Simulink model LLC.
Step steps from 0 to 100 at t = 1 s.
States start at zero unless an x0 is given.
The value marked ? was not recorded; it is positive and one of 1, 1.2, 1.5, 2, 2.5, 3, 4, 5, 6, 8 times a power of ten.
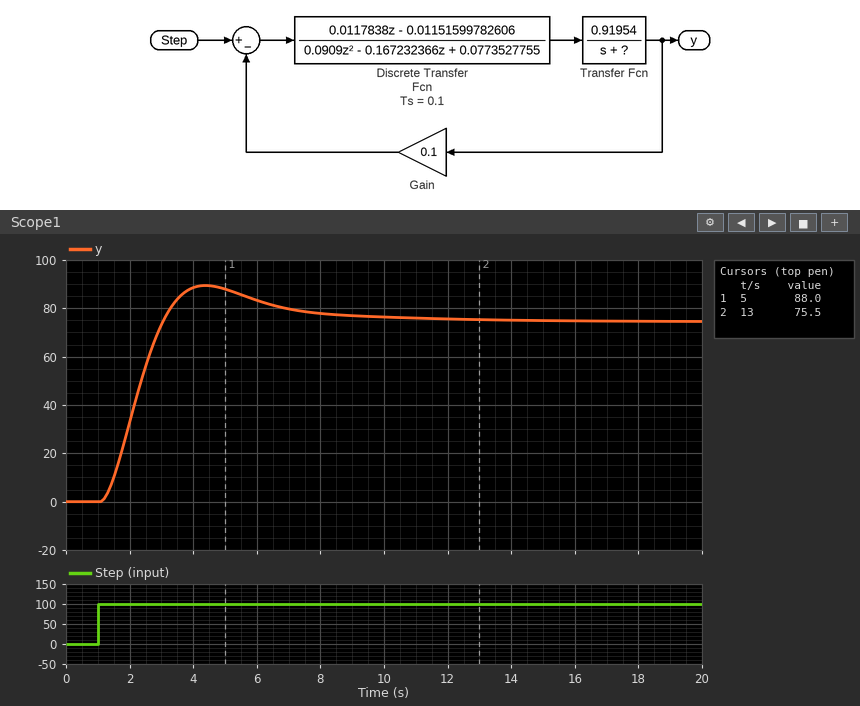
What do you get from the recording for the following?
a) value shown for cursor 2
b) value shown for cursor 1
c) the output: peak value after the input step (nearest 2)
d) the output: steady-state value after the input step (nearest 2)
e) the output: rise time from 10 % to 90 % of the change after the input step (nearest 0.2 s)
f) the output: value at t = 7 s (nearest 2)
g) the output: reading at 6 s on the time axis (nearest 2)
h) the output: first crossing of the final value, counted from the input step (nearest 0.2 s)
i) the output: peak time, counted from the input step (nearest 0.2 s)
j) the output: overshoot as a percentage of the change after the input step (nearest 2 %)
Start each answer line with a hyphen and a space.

- 75.5
- 88.0
- 90
- 74
- 1.4 s
- 80
- 84
- 2.0 s
- 3.4 s
- 20 %
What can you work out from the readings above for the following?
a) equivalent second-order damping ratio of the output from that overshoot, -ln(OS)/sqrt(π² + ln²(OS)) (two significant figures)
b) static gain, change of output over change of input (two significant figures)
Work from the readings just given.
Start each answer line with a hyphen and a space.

- 0.46
- 0.74
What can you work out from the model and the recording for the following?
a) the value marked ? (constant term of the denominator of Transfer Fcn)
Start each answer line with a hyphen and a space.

- 0.3
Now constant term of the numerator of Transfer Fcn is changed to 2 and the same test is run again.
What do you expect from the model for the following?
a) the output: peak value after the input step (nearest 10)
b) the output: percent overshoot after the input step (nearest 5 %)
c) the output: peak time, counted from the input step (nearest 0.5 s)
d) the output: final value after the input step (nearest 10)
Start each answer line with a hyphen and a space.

- 180
- 20 %
- 3.0 s
- 150
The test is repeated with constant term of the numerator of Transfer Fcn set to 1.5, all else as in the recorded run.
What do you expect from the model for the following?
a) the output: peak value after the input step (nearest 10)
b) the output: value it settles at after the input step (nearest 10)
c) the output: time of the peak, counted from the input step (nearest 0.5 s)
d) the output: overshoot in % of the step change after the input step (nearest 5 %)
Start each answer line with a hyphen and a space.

- 140
- 120
- 3.0 s
- 20 %
